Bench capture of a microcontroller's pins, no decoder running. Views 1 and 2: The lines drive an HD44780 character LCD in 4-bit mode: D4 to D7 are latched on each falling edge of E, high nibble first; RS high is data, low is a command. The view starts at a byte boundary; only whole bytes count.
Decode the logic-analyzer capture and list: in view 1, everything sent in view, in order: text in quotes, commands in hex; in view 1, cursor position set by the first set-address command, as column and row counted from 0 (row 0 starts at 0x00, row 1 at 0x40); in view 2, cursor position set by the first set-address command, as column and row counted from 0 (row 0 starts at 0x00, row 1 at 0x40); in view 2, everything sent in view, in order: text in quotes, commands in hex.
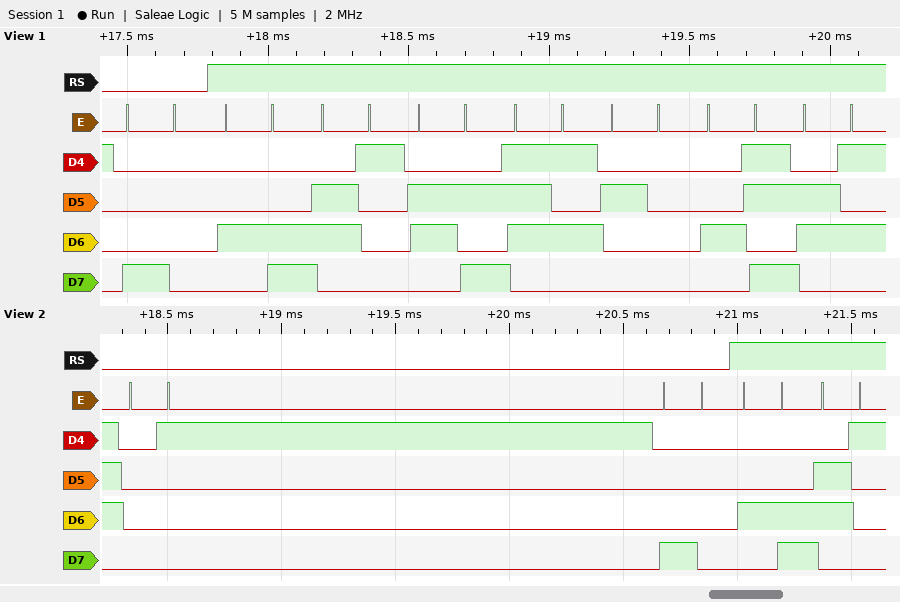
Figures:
0x80 "Laju Ke"
column 0, row 0
column 0, row 0
0x01 0x80 "La"
